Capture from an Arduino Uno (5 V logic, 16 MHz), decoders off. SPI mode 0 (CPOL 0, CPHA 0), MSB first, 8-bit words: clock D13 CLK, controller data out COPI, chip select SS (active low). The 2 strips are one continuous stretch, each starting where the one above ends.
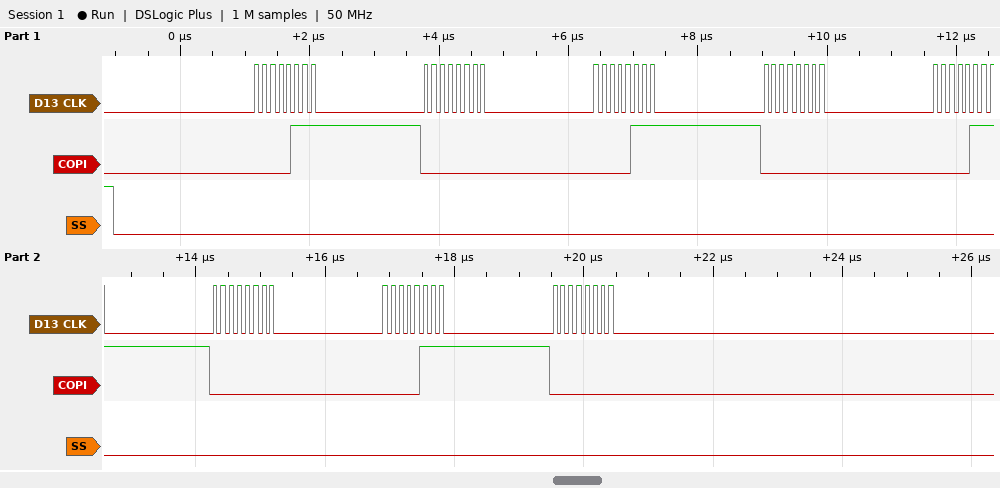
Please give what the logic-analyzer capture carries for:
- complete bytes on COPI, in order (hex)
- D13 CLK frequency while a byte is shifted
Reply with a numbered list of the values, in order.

1. 0x07 0x00 0x07 0x00 0x07 0x00 0x07 0x00
2. 8 MHz
